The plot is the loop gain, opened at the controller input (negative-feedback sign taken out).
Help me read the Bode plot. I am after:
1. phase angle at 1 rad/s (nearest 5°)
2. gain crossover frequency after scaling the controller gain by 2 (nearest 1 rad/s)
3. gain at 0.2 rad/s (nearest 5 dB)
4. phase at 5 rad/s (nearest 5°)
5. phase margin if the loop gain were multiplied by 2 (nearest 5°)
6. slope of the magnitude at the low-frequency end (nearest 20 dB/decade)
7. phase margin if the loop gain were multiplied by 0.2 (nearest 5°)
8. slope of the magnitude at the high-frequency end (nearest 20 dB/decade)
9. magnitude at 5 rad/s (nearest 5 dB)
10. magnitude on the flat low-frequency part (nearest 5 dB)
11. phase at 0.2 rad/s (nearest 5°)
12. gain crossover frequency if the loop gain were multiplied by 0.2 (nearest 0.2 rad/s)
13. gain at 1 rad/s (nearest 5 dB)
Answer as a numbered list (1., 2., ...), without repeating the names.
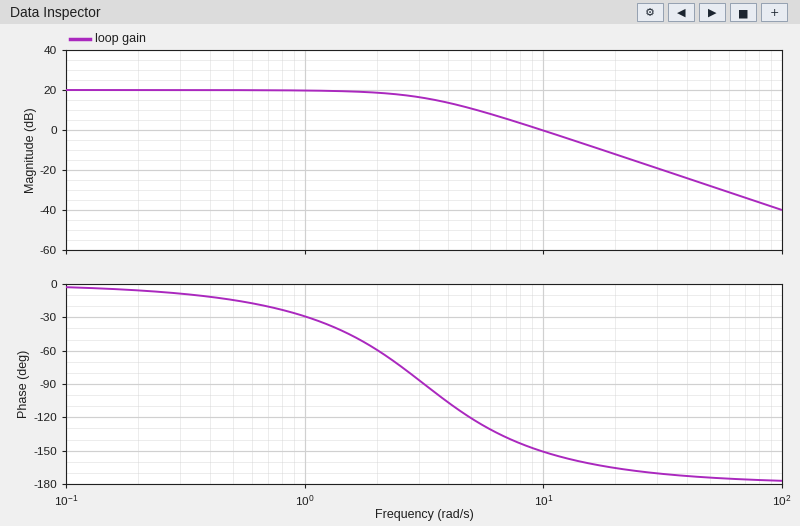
1. -30°
2. 14 rad/s
3. 20 dB
4. -120°
5. 20°
6. 0 dB/decade
7. 75°
8. -40 dB/decade
9. 10 dB
10. 20 dB
11. -5°
12. 3.8 rad/s
13. 20 dB
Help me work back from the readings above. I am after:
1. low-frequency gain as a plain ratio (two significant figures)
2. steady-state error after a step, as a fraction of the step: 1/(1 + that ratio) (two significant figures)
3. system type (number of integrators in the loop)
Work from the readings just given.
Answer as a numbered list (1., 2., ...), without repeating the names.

1. 10
2. 0.091
3. 0
